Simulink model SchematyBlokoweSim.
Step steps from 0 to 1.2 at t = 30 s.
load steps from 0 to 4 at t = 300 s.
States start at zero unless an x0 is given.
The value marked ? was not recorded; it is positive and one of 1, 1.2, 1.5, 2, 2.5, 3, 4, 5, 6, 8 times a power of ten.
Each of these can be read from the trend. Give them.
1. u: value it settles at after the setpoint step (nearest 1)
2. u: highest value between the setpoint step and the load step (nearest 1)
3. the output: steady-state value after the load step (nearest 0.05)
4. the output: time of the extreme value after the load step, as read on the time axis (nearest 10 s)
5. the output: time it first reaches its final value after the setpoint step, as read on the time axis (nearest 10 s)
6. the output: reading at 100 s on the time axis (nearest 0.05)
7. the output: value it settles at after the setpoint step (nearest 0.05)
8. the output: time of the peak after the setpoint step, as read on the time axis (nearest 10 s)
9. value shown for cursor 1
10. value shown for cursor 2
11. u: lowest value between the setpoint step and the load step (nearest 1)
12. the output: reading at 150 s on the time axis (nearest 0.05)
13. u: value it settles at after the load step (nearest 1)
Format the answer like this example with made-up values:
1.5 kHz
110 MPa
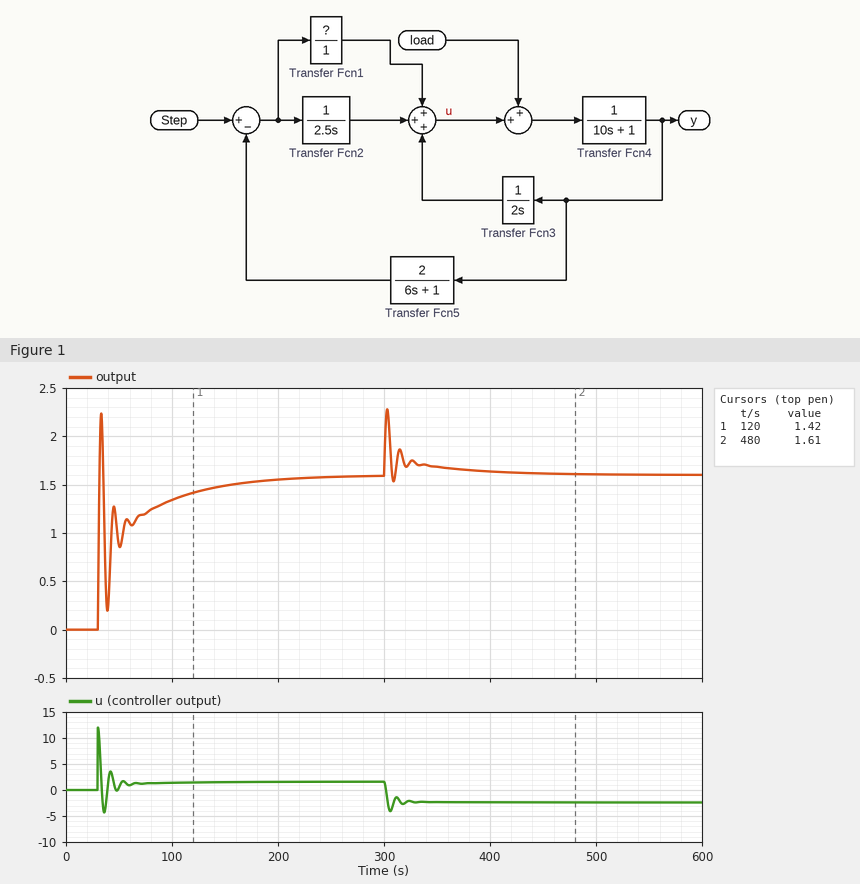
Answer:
2
12
1.60
300 s
30 s
1.35
1.60
30 s
1.42
1.61
-4
1.50
-2
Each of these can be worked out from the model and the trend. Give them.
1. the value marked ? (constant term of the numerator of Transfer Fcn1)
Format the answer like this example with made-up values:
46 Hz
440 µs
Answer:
10
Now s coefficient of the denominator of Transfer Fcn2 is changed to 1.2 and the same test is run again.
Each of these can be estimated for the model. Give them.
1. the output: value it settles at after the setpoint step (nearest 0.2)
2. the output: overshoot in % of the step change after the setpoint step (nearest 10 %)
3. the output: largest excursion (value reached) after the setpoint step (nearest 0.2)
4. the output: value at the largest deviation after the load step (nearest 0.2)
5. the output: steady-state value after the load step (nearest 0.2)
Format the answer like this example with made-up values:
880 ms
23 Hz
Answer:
0.8
180 %
2.4
1.6
0.8
